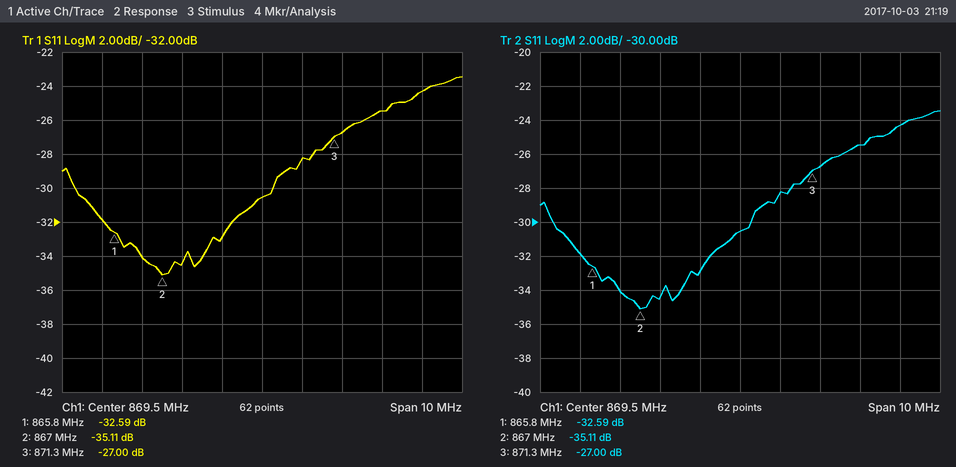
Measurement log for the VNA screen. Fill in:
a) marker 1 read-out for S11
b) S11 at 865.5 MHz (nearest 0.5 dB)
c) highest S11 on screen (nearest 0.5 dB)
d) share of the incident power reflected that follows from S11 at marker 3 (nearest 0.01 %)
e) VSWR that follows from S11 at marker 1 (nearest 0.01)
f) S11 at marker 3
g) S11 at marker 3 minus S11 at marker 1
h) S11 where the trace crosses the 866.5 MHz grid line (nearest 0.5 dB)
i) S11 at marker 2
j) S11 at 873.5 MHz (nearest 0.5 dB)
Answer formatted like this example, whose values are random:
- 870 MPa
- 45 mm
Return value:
- -32.59 dB
- -32.0 dB
- -23.5 dB
- 0.20 %
- 1.05
- -27.00 dB
- 5.59 dB
- -34.0 dB
- -35.11 dB
- -24.5 dB
